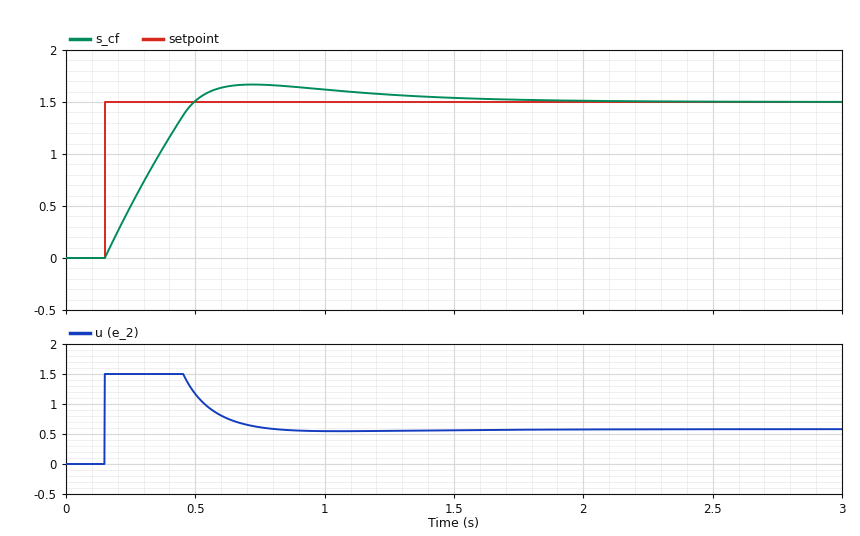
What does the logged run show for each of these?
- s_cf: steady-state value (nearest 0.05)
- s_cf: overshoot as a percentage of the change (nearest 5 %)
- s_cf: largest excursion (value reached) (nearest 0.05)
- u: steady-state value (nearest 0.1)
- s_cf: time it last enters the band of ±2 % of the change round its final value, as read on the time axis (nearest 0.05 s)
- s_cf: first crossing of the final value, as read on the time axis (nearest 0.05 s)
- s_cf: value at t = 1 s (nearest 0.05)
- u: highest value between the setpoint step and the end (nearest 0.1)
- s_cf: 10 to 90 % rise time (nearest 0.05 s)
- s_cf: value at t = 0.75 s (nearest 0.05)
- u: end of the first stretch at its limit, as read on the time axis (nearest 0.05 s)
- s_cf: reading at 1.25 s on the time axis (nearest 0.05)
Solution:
1.50
10 %
1.65
0.6
1.60 s
0.50 s
1.60
1.5
0.25 s
1.65
0.45 s
1.55
